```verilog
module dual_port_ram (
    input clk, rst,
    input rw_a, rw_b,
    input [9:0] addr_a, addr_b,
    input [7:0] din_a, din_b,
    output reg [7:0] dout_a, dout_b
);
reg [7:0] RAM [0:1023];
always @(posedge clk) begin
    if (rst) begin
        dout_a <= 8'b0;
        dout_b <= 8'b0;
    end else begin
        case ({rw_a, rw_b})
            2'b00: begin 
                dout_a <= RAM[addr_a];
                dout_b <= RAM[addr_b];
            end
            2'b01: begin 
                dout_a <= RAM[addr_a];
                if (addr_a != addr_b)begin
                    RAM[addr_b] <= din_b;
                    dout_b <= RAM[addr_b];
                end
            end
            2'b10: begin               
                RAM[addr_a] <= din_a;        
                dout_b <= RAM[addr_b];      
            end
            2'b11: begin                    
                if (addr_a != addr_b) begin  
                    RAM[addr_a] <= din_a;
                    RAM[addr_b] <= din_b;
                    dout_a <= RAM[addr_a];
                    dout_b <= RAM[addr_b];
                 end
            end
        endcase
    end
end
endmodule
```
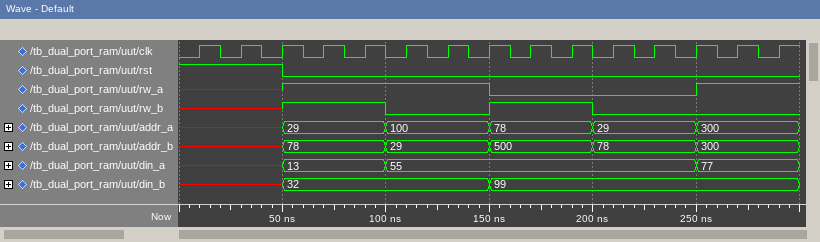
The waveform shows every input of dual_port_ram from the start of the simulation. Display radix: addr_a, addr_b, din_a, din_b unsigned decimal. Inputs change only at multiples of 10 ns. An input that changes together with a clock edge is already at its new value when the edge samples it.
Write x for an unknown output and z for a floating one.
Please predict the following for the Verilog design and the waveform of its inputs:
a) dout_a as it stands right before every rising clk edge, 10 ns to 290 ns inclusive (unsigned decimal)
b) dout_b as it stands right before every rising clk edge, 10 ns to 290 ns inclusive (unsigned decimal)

x, 0, 0, x, 13, 13, 13, 13, 32, 32, 32, 13, 13, 13, 13
x, 0, 0, x, 32, 32, 13, 13, x, 99, 99, 32, 32, x, 77
